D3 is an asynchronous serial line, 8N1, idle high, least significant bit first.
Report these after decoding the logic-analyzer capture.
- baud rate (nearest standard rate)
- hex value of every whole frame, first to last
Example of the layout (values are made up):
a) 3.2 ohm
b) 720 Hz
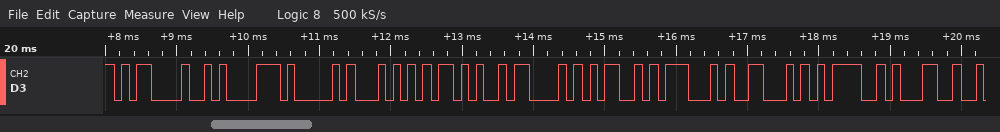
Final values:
a) 9600 baud
b) 0x0D 0x0A 0x41 0x54 0x2B 0x43 0x4D 0x47 0x46 0x3D 0x31
